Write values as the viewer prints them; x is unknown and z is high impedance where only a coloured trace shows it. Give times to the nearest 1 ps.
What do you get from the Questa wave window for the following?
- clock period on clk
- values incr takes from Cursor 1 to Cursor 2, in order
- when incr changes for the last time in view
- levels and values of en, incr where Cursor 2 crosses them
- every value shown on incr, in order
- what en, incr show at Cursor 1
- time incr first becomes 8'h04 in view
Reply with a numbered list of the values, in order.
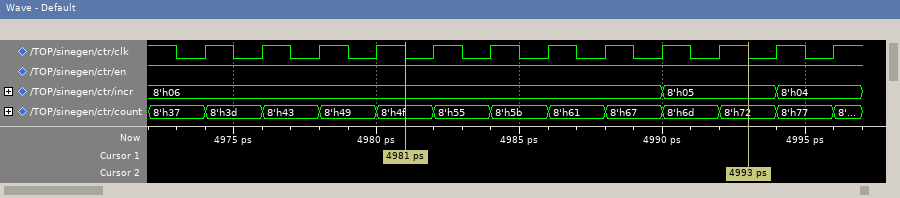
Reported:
1. 2 ps
2. 8'h06, 8'h05
3. 4994 ps
4. en=1, incr=8'h05
5. 8'h06, 8'h05, 8'h04
6. en=1, incr=8'h06
7. 4994 ps
